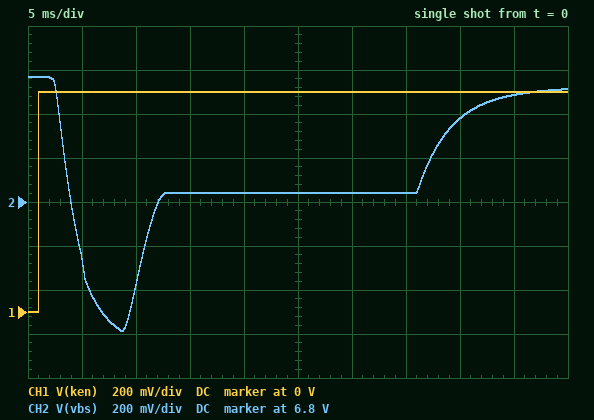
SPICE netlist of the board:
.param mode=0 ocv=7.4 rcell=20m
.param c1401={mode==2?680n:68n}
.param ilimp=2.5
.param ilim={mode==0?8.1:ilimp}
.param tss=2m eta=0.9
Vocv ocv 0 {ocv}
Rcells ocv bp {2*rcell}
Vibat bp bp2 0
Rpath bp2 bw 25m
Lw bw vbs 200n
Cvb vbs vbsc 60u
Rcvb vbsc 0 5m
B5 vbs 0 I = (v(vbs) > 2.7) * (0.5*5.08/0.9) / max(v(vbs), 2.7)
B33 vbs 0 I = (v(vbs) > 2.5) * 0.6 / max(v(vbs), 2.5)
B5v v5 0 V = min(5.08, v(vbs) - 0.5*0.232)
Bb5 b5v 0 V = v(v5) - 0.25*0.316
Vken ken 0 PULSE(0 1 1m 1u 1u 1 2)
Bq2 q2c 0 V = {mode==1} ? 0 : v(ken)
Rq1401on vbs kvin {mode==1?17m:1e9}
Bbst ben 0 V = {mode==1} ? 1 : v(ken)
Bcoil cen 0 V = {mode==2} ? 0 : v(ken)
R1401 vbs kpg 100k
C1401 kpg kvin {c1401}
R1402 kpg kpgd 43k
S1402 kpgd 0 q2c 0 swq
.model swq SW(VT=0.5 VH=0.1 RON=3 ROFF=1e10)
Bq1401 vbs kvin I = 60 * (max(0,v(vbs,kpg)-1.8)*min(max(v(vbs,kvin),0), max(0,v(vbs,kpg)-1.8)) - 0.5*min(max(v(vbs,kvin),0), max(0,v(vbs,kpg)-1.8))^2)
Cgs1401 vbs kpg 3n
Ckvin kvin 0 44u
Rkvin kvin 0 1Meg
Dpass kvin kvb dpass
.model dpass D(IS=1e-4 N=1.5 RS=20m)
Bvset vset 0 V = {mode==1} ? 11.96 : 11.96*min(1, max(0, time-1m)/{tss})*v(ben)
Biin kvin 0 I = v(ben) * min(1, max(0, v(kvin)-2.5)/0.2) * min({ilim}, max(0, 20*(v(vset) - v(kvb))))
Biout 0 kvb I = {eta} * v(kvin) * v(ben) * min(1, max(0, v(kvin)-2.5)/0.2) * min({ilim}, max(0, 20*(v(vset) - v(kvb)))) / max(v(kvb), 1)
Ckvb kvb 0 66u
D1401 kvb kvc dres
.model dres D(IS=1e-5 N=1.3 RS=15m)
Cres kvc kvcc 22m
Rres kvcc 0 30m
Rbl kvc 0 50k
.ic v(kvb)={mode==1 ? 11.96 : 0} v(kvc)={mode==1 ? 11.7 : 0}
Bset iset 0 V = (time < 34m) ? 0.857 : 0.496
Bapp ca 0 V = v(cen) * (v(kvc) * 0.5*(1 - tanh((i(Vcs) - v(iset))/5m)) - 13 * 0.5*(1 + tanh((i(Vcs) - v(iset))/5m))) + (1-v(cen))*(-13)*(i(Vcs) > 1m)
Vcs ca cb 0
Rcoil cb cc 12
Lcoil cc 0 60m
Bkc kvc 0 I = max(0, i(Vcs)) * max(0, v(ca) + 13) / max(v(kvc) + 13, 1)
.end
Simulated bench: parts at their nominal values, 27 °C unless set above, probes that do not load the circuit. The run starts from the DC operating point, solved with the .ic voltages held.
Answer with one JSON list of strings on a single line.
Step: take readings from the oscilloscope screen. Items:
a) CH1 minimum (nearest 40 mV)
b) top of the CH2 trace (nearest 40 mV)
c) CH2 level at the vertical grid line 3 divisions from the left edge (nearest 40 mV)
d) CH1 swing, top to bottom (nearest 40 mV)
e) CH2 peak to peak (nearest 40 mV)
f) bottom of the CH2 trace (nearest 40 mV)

["0 V", "7.36 V", "6.84 V", "1.00 V", "1.16 V", "6.20 V"]
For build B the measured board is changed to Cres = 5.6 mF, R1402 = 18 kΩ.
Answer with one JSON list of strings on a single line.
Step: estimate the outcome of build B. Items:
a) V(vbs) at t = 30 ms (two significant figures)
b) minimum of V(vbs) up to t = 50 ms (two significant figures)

["7.3 V", "6.4 V"]
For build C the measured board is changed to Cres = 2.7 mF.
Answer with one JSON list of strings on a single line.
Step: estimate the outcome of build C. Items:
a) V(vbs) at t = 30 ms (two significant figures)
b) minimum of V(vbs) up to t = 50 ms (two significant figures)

["7.3 V", "6.8 V"]
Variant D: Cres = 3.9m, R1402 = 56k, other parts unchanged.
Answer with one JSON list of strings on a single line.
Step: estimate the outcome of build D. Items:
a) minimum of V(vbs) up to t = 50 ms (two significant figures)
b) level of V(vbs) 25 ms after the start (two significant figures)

["6.8 V", "7.3 V"]
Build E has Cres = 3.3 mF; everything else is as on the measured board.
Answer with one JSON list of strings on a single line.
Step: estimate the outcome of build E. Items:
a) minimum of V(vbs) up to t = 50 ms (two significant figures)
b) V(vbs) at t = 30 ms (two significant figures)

["6.8 V", "7.3 V"]
